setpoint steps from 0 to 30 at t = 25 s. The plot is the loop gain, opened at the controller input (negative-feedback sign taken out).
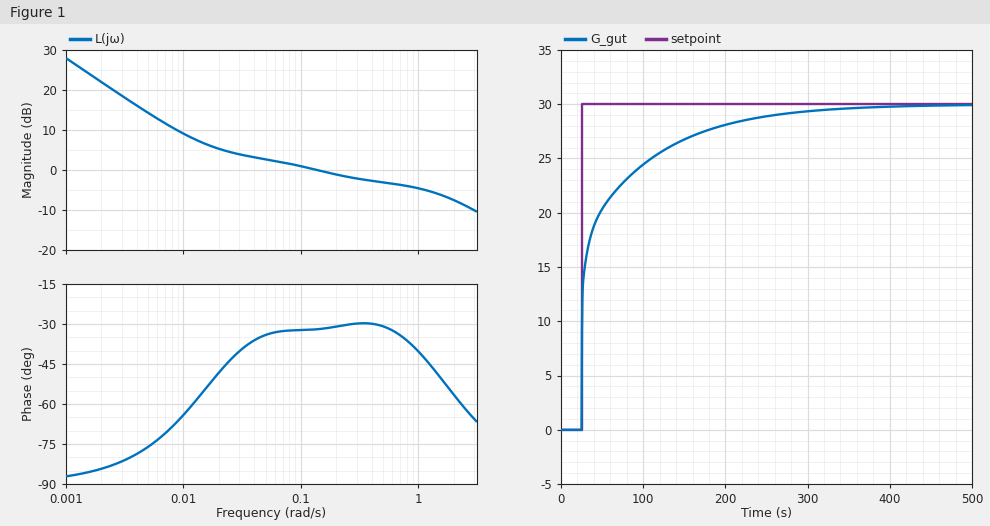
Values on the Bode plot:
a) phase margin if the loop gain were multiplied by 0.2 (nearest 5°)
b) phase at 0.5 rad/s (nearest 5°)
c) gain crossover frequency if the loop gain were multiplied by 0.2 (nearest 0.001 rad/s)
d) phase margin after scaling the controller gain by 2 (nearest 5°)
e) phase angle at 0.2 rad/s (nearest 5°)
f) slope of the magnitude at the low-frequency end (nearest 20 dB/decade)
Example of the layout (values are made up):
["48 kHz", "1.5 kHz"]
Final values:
["105°", "-30°", "0.005 rad/s", "130°", "-30°", "-20 dB/decade"]
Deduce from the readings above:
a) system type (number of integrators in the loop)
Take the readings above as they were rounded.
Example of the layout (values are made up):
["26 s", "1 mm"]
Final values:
["1"]
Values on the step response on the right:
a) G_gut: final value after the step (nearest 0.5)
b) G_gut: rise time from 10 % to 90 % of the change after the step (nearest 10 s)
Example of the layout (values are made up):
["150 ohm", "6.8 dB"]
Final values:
["30.0", "130 s"]
